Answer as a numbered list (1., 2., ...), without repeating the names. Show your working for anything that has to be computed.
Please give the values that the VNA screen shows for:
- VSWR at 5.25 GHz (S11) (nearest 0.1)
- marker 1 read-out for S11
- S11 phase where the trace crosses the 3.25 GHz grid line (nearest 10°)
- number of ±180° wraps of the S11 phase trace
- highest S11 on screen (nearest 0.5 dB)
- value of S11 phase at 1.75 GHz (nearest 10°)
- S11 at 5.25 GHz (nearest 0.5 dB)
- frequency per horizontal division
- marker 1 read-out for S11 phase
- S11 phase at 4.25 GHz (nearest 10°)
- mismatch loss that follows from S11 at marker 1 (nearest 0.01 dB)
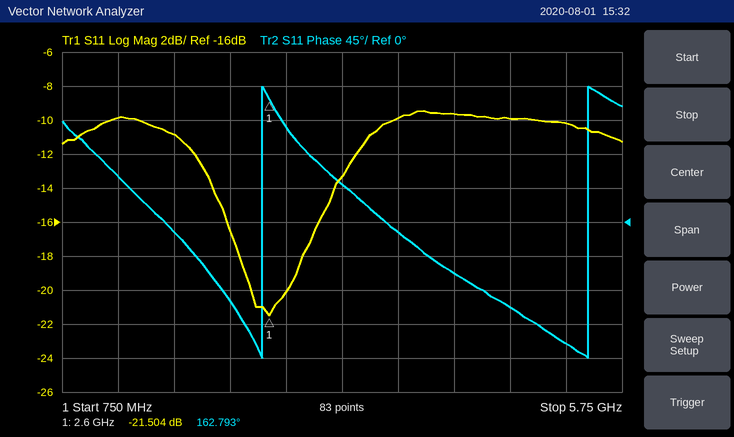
1. |Γ| = 10^(-10/20) = 0.3162; VSWR = (1 + 0.3162)/(1 − 0.3162) ≈ 1.9
2. -21.504 dB
3. 50°
4. 2
5. -9.5 dB
6. -10°
7. -10.0 dB
8. 500 MHz
9. 162.793°
10. -70°
11. −10 log10(1 − 10^(-21.504/10)) ≈ 0.03 dB
